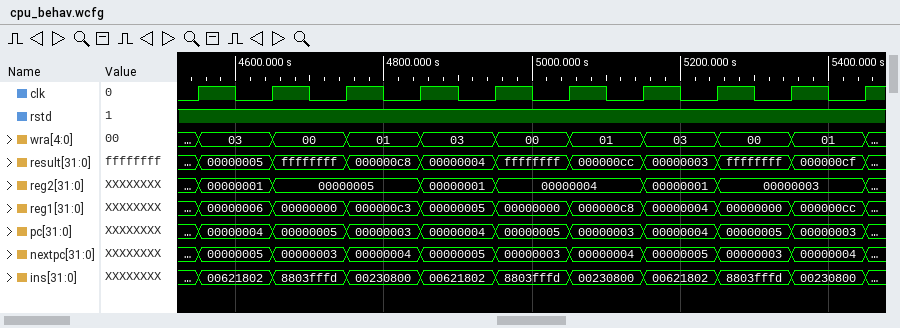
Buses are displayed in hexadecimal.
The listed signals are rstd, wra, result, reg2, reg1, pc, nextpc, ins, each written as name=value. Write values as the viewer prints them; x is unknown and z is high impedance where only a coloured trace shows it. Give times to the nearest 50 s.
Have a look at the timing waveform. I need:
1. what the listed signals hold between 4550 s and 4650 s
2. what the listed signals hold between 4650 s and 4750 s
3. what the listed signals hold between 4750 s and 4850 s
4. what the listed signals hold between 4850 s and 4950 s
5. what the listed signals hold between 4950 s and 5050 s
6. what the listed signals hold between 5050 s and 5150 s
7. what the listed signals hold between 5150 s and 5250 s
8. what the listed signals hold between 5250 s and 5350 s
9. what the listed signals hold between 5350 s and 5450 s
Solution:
rstd=1, wra=03, result=00000005, reg2=00000001, reg1=00000006, pc=00000004, nextpc=00000005, ins=00621802
rstd=1, wra=00, result=ffffffff, reg2=00000005, reg1=00000000, pc=00000005, nextpc=00000003, ins=8803fffd
rstd=1, wra=01, result=000000c8, reg2=00000005, reg1=000000c3, pc=00000003, nextpc=00000004, ins=00230800
rstd=1, wra=03, result=00000004, reg2=00000001, reg1=00000005, pc=00000004, nextpc=00000005, ins=00621802
rstd=1, wra=00, result=ffffffff, reg2=00000004, reg1=00000000, pc=00000005, nextpc=00000003, ins=8803fffd
rstd=1, wra=01, result=000000cc, reg2=00000004, reg1=000000c8, pc=00000003, nextpc=00000004, ins=00230800
rstd=1, wra=03, result=00000003, reg2=00000001, reg1=00000004, pc=00000004, nextpc=00000005, ins=00621802
rstd=1, wra=00, result=ffffffff, reg2=00000003, reg1=00000000, pc=00000005, nextpc=00000003, ins=8803fffd
rstd=1, wra=01, result=000000cf, reg2=00000003, reg1=000000cc, pc=00000003, nextpc=00000004, ins=00230800
